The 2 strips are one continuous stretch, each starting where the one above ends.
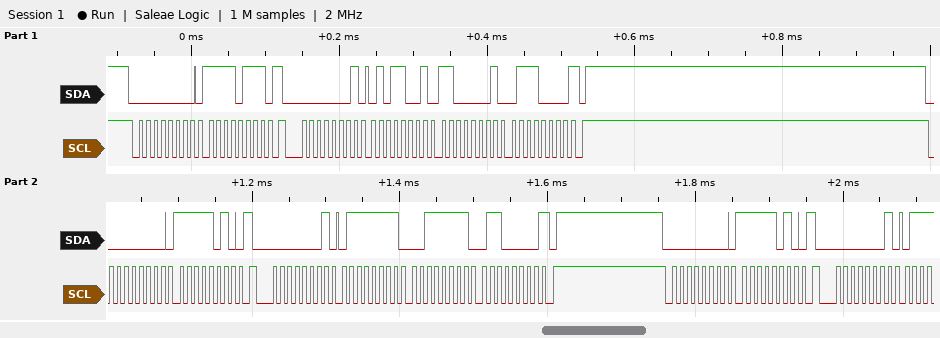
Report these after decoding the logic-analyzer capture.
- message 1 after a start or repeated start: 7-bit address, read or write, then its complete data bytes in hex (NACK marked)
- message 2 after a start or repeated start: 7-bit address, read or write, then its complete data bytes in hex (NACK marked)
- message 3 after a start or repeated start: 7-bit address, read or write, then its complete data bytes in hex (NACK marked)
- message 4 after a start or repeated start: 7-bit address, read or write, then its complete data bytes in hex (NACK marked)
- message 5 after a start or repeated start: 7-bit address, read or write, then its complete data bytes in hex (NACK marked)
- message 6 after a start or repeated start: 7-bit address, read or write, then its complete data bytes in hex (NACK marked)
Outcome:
0x00 write: F7
0x00 read: 59 C1 70 NACK
0x00 write: FA
0x00 read: 7F 3F 60 NACK
0x00 write: FA
0x00 read
